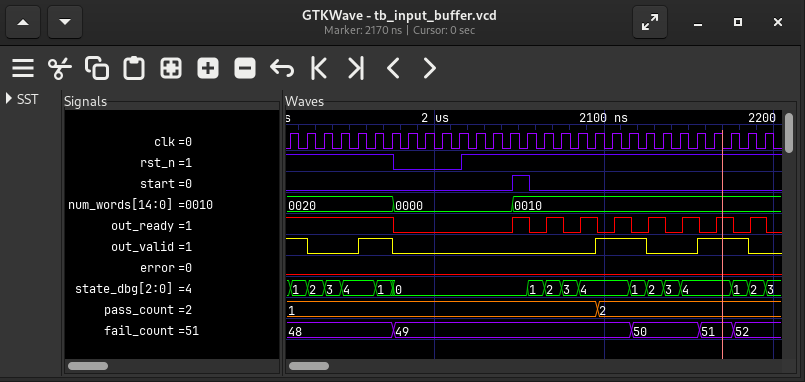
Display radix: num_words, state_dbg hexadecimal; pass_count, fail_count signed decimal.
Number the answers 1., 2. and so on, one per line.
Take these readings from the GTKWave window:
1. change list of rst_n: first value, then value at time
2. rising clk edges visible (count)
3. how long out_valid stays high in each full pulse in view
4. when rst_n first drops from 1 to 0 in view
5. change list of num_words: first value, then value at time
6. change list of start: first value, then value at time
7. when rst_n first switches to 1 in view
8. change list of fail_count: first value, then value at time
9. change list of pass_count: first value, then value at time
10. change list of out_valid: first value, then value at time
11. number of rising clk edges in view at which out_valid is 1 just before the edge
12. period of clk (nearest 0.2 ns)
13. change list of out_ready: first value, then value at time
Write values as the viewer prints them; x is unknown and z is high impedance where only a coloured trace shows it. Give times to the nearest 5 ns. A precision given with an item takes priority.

1. 1, 0 at 1975 ns, 1 at 2015 ns
2. 29
3. 20 ns, 30 ns, 30 ns
4. 1975 ns
5. 0020, 0000 at 1975 ns, 0010 at 2045 ns
6. 0, 1 at 2045 ns, 0 at 2055 ns
7. 2015 ns
8. 48, 49 at 1975 ns, 50 at 2115 ns, 51 at 2155 ns, 52 at 2175 ns
9. 1, 2 at 2095 ns
10. 1, 0 at 1925 ns, 1 at 1955 ns, 0 at 1975 ns, 1 at 2095 ns, 0 at 2125 ns, 1 at 2155 ns, 0 at 2185 ns
11. 10
12. 10 ns
13. 1, 0 at 1975 ns, 1 at 2045 ns, 0 at 2055 ns, 1 at 2065 ns, 0 at 2075 ns, 1 at 2085 ns, 0 at 2095 ns, 1 at 2105 ns, 0 at 2115 ns, 1 at 2125 ns, 0 at 2135 ns, 1 at 2145 ns, 0 at 2155 ns, 1 at 2165 ns, 0 at 2175 ns, 1 at 2185 ns, 0 at 2195 ns
